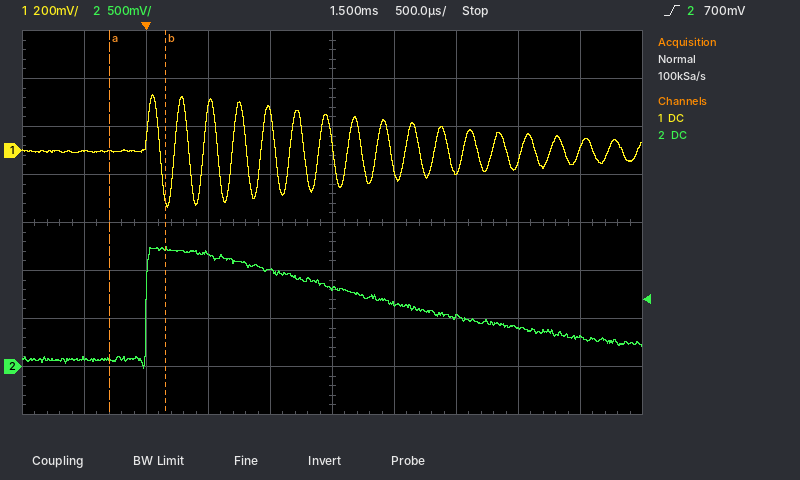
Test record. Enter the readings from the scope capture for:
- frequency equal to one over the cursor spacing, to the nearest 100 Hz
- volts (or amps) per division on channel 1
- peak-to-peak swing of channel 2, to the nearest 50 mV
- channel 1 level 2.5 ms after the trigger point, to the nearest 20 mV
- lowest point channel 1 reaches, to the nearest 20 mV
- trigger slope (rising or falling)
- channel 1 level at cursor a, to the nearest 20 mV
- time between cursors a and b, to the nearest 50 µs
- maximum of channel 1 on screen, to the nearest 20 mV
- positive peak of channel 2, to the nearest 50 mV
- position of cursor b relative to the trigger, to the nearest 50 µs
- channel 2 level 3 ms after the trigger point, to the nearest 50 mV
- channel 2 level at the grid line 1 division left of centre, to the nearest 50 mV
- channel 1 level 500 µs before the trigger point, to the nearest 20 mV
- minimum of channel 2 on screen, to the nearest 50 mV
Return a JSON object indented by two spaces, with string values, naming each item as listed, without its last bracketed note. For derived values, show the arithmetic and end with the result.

{
  "frequency equal to one over the cursor spacing, to the nearest 100 Hz": "1 / 450 µs ≈ 2.2 kHz",
  "volts (or amps) per division on channel 1": "200 mV",
  "peak-to-peak swing of channel 2, to the nearest 50 mV": "1.25 V − (0 mV) = 1.25 V",
  "channel 1 level 2.5 ms after the trigger point, to the nearest 20 mV": "-80 mV",
  "lowest point channel 1 reaches, to the nearest 20 mV": "-240 mV",
  "trigger slope": "rising",
  "channel 1 level at cursor a, to the nearest 20 mV": "0 mV",
  "time between cursors a and b, to the nearest 50 µs": "450 µs",
  "maximum of channel 1 on screen, to the nearest 20 mV": "240 mV",
  "positive peak of channel 2, to the nearest 50 mV": "1.25 V",
  "position of cursor b relative to the trigger, to the nearest 50 µs": "+150 µs",
  "channel 2 level 3 ms after the trigger point, to the nearest 50 mV": "400 mV",
  "channel 2 level at the grid line 1 division left of centre, to the nearest 50 mV": "1.00 V",
  "channel 1 level 500 µs before the trigger point, to the nearest 20 mV": "0 mV",
  "minimum of channel 2 on screen, to the nearest 50 mV": "0 mV"
}
